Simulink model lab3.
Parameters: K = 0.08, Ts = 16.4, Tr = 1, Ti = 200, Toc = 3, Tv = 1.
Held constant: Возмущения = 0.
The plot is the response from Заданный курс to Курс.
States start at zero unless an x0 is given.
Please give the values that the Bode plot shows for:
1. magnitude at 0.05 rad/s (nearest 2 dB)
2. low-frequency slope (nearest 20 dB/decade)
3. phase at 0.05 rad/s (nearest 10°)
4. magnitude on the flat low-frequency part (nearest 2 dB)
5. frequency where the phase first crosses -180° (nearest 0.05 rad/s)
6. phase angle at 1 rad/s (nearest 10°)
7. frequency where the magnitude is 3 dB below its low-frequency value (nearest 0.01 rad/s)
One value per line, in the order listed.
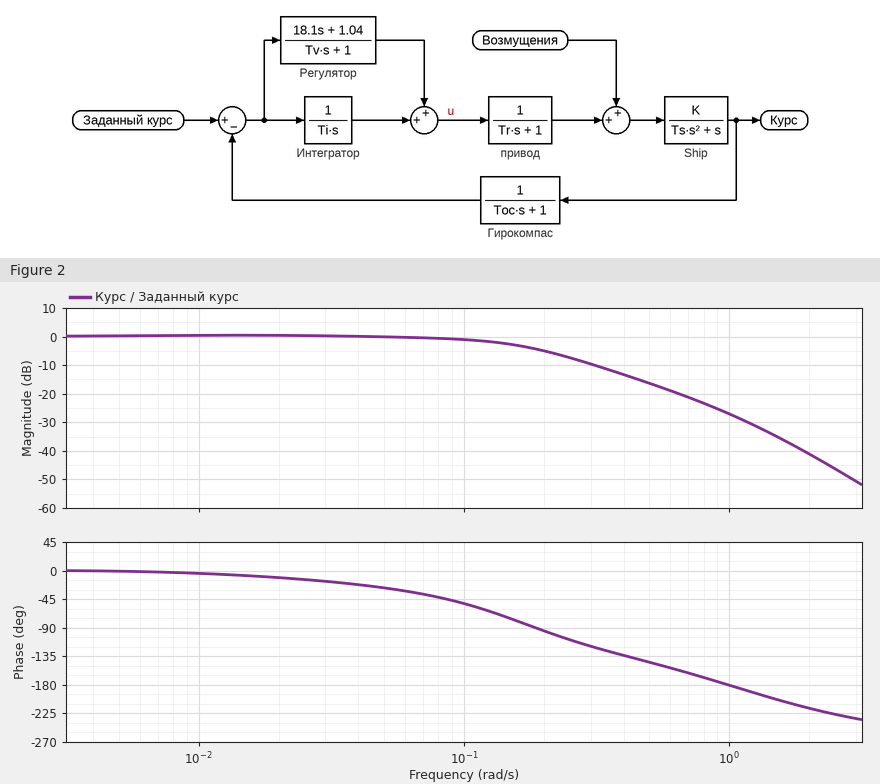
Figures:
0 dB
0 dB/decade
-30°
0 dB
1.00 rad/s
-180°
0.15 rad/s
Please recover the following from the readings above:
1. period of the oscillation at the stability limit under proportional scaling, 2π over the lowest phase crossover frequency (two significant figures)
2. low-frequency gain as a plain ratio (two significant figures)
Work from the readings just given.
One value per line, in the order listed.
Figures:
6.3 s
1.0
